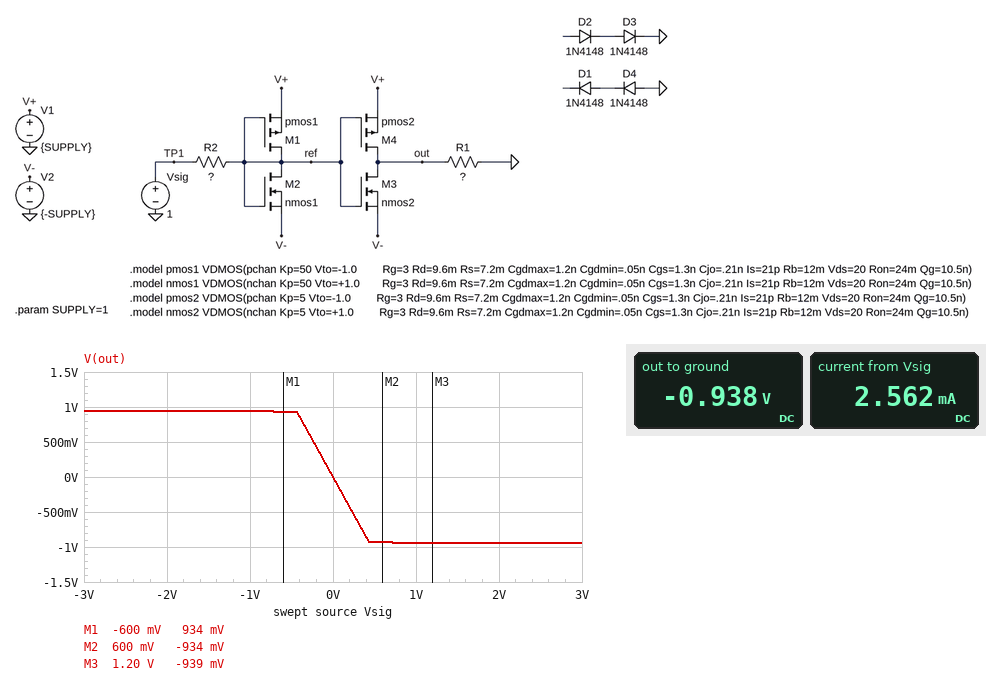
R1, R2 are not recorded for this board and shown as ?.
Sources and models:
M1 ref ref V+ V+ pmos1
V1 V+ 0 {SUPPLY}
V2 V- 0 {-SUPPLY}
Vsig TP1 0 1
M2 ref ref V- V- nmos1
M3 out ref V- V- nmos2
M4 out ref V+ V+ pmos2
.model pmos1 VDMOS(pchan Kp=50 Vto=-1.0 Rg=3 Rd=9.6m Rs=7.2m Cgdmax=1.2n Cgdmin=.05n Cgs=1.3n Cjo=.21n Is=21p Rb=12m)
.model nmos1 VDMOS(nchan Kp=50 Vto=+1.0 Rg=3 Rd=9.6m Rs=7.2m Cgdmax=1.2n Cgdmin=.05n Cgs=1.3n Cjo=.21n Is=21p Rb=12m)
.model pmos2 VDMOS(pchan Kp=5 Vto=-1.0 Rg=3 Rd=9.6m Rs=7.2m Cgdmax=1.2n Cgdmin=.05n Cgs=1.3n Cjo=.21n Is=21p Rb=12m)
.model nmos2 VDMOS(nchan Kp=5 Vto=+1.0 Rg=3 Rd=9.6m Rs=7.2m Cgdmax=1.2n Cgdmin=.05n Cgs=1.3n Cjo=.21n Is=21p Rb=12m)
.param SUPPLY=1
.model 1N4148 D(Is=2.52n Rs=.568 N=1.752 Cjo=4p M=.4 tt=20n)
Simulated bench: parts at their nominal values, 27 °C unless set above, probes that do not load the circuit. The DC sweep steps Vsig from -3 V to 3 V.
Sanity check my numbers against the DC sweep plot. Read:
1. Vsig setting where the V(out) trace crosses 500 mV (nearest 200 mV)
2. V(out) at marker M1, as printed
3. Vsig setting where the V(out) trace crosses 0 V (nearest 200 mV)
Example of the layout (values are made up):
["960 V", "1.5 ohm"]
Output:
["-200 mV", "934 mV", "0 V"]
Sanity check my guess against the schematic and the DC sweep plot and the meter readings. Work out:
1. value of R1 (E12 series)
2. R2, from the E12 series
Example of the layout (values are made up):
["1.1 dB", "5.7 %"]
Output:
["8.2 kΩ", "390 Ω"]
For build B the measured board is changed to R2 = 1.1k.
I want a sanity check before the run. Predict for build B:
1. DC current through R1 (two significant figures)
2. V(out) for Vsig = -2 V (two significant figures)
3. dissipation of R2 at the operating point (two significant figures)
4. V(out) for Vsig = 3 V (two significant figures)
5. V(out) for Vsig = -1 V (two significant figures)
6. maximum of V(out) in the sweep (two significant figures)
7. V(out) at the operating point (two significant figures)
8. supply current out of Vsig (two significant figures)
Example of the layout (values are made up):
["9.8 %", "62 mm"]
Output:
["93 µA", "940 mV", "910 µW", "-940 mV", "760 mV", "940 mV", "-760 mV", "910 µA"]
